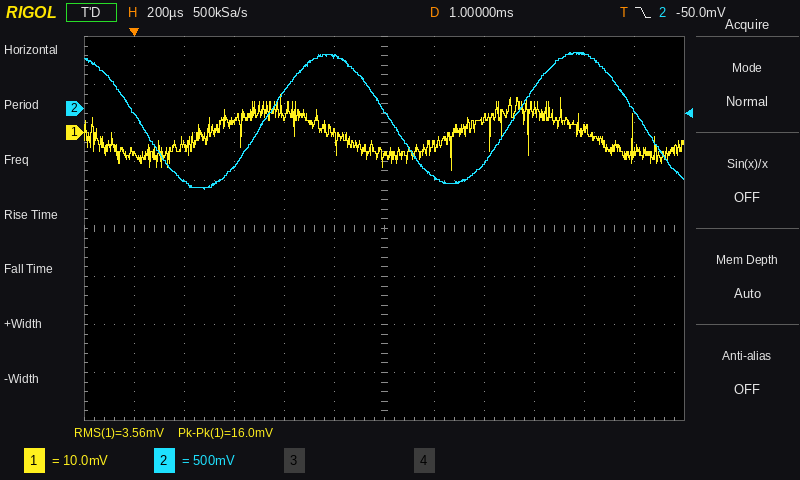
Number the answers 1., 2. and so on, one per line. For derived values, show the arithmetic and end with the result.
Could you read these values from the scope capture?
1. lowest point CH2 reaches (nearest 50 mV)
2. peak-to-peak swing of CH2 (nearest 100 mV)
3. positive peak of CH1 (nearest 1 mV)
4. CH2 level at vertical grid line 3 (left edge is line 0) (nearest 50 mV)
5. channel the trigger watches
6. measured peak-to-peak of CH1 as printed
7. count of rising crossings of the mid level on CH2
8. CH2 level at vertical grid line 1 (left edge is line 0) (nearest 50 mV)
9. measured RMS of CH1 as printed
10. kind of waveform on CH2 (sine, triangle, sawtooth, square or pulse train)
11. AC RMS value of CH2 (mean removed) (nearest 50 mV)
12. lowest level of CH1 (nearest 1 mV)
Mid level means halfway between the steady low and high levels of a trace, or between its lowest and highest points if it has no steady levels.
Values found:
1. -850 mV
2. 1.40 V
3. 8 mV
4. -600 mV
5. CH2
6. 16.0 mV
7. 2
8. -50 mV
9. 3.56 mV
10. sine
11. 1.40 V / (2√2) ≈ 495 mV, so 500 mV to the nearest 50 mV
12. -8 mV
